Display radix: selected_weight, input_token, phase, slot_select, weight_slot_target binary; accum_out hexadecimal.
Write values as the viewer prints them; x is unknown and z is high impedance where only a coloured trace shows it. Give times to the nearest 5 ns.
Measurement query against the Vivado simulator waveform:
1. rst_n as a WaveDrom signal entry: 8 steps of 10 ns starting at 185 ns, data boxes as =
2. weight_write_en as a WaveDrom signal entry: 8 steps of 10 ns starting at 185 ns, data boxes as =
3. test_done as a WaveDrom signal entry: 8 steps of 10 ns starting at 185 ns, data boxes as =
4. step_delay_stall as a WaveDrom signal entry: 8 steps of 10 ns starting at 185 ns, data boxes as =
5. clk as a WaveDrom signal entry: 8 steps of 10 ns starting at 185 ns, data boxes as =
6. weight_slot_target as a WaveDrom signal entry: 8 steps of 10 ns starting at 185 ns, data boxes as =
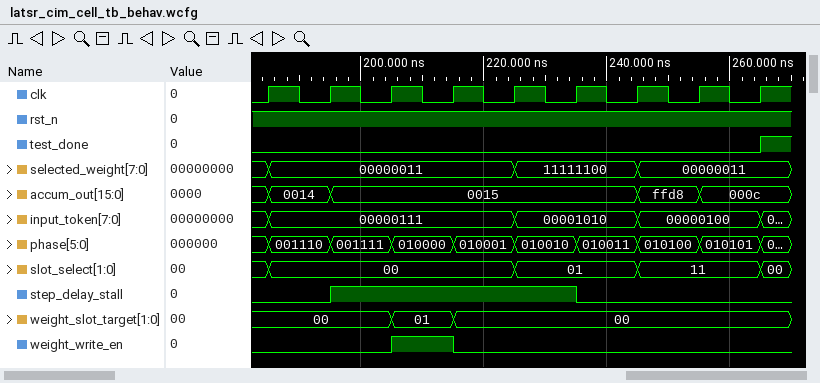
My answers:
{name: 'rst_n', wave: '1.......'}
{name: 'weight_write_en', wave: '0.10....'}
{name: 'test_done', wave: '0.......'}
{name: 'step_delay_stall', wave: '01...0..'}
{name: 'clk', wave: 'p.......'}
{name: 'weight_slot_target', wave: '=.==....', data: '00 01 00'}
